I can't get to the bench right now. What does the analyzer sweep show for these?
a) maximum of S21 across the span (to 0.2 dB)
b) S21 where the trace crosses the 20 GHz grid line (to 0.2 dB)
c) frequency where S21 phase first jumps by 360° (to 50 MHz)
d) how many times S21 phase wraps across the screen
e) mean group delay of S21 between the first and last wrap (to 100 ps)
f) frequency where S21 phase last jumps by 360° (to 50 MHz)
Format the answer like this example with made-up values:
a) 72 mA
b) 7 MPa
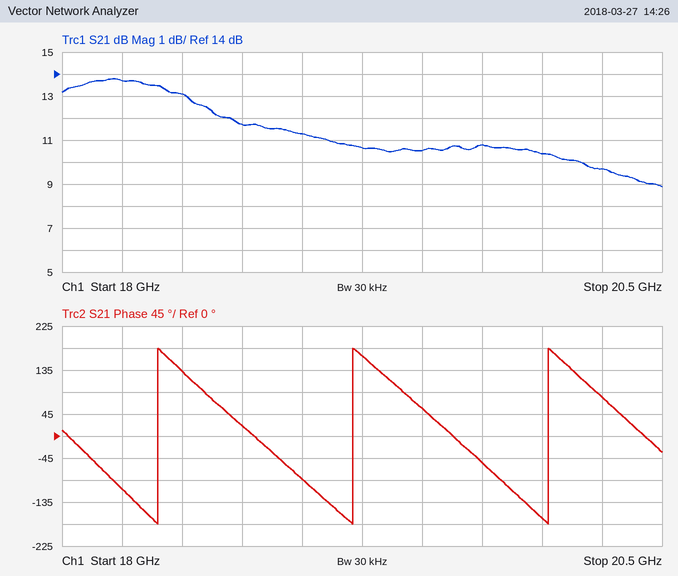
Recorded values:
a) 13.8 dB
b) 10.4 dB
c) 18.40 GHz
d) 3
e) 1.2 ns
f) 20.05 GHz
